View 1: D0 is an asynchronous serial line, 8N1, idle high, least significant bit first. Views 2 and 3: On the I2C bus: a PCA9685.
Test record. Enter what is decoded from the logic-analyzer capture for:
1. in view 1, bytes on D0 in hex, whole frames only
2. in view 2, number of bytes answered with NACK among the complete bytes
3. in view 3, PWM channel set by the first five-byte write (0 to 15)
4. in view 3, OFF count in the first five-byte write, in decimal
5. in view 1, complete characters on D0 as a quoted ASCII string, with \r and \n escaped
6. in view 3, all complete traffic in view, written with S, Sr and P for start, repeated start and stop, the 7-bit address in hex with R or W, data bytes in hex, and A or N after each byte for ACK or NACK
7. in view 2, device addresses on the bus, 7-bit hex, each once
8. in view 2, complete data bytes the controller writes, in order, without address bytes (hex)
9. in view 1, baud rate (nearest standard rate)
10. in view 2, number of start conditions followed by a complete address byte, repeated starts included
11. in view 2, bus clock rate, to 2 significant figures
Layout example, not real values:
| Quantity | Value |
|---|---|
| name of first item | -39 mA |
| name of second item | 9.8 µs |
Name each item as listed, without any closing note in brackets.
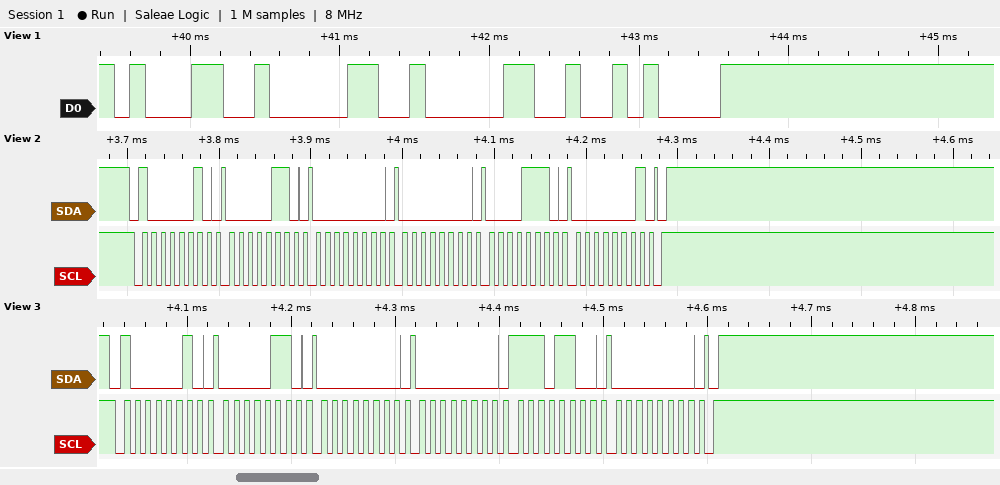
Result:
| Quantity | Value |
|---|---|
| in view 1, bytes on D0 in hex, whole frames only | 31 30 30 0A |
| in view 2, number of bytes answered with NACK among the complete bytes | 0 |
| in view 3, PWM channel set by the first five-byte write | 0 |
| in view 3, OFF count in the first five-byte write, in decimal | 236 |
| in view 1, complete characters on D0 as a quoted ASCII string, with \r and \n escaped | "100\n" |
| in view 3, all complete traffic in view, written with S, Sr and P for start, repeated start and stop, the 7-bit address in hex with R or W, data bytes in hex, and A or N after each byte for ACK or NACK | S 41W A 06 A 00 A 00 A EC A 00 A P |
| in view 2, device addresses on the bus, 7-bit hex, each once | 0x41 |
| in view 2, complete data bytes the controller writes, in order, without address bytes | 06 00 00 0E 01 |
| in view 1, baud rate | 9600 baud |
| in view 2, number of start conditions followed by a complete address byte, repeated starts included | 1 |
| in view 2, bus clock rate, to 2 significant figures | 100 kHz |
